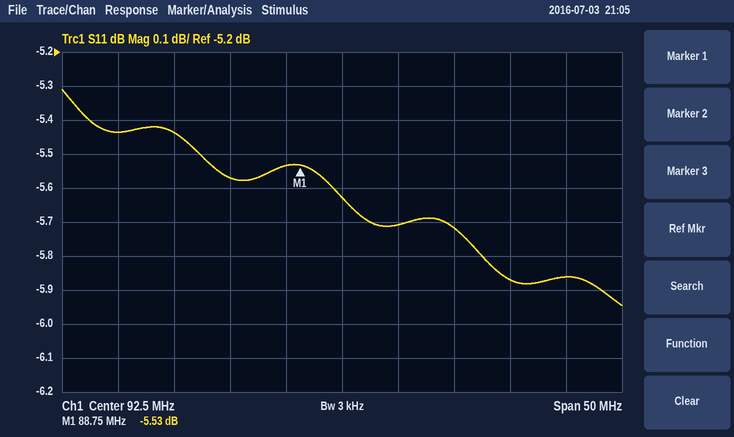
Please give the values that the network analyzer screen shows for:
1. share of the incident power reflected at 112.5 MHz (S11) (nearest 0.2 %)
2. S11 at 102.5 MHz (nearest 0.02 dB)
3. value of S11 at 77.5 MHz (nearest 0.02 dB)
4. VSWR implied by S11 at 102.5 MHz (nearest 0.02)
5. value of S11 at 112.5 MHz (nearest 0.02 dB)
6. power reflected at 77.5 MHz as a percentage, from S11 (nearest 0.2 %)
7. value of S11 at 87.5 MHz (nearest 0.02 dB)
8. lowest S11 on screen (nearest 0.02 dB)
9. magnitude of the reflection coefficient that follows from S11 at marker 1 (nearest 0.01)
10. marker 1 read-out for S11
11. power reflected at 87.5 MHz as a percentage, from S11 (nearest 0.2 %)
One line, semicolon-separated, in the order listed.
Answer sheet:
26.0 %; -5.72 dB; -5.44 dB; 3.14; -5.86 dB; 28.6 %; -5.54 dB; -5.94 dB; 0.53; -5.53 dB; 28.0 %
